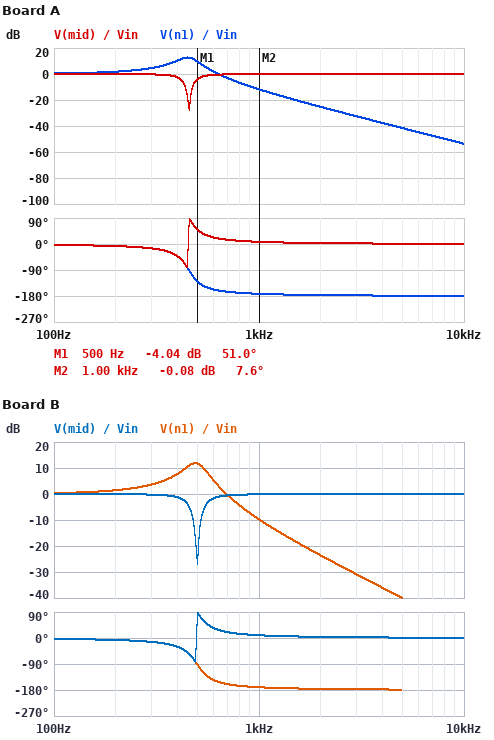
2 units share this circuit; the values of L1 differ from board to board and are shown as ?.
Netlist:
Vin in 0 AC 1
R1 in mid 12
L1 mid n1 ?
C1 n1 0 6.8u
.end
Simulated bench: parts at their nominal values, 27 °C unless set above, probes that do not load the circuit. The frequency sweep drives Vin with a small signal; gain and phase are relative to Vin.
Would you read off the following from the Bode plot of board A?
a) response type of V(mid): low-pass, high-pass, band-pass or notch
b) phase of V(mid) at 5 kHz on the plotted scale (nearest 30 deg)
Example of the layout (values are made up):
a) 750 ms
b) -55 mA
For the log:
a) notch
b) 0 deg
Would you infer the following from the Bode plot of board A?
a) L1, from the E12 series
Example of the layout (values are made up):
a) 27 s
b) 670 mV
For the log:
a) 18 mH
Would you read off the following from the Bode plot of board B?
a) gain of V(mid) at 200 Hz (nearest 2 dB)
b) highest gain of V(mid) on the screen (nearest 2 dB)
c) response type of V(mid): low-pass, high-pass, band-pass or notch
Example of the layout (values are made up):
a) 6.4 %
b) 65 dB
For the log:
a) 0 dB
b) 0 dB
c) notch
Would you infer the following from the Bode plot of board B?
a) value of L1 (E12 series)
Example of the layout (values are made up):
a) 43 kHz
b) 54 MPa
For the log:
a) 15 mH
